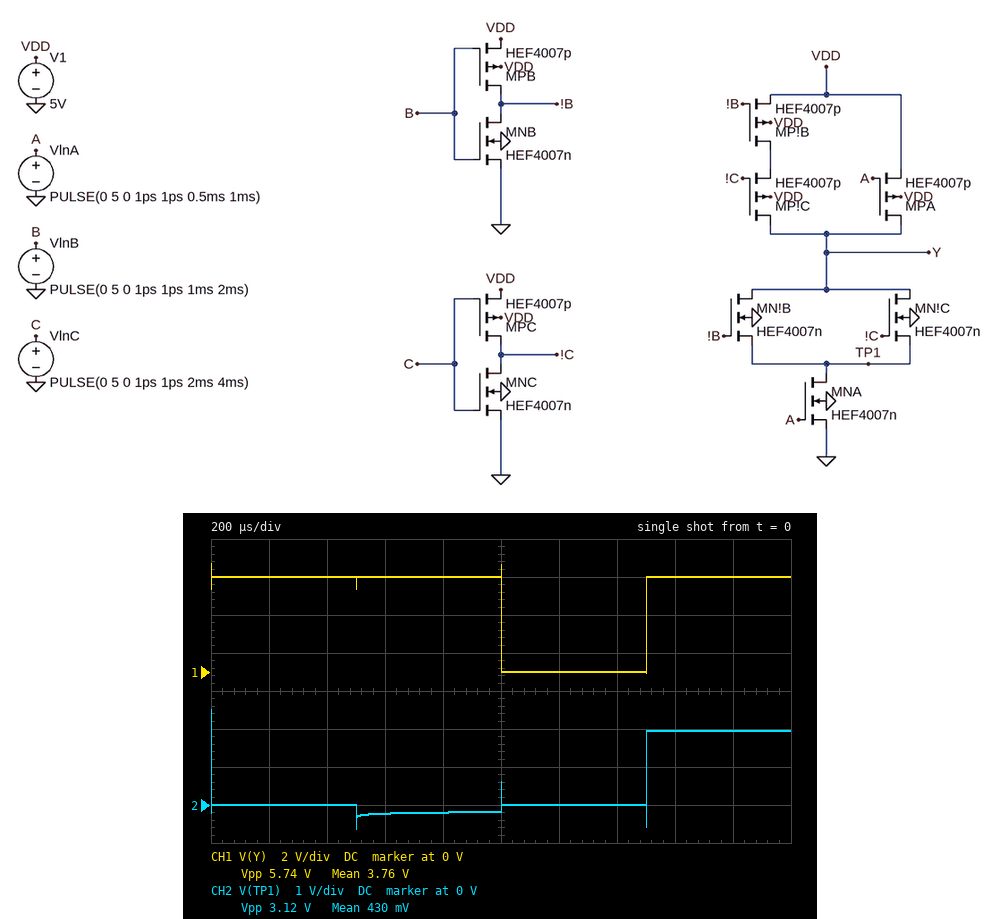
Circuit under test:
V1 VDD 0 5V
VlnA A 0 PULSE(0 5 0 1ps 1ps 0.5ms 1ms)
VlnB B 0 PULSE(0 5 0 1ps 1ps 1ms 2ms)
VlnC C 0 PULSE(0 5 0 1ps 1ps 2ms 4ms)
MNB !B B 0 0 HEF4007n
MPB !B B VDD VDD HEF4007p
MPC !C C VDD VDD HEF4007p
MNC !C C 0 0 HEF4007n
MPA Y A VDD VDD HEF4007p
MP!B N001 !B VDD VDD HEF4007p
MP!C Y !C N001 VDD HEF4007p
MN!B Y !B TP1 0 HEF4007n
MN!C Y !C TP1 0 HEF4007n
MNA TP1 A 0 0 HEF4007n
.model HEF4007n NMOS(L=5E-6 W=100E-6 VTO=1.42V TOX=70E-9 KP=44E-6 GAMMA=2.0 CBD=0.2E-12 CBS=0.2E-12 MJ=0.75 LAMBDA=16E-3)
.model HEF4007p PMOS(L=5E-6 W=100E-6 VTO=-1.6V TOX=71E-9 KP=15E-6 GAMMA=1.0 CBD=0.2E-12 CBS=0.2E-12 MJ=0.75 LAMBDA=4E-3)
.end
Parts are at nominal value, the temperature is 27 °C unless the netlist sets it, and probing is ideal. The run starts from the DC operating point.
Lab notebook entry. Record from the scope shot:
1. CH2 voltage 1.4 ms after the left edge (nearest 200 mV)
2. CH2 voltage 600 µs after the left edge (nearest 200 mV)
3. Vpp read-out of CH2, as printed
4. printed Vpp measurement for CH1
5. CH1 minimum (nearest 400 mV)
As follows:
0 V
-200 mV
3.12 V
5.74 V
0 V
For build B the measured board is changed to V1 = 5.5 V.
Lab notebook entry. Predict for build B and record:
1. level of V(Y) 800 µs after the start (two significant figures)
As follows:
5.5 V
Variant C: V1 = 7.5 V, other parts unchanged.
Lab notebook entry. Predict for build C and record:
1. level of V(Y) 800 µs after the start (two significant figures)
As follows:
7.5 V
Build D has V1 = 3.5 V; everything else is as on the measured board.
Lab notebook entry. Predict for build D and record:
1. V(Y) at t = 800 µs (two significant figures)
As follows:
3.5 V
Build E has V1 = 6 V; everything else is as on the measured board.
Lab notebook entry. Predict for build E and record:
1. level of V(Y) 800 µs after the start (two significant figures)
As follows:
6.0 V
